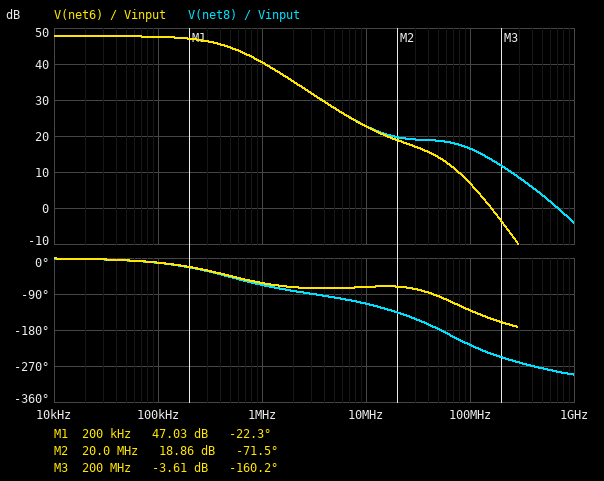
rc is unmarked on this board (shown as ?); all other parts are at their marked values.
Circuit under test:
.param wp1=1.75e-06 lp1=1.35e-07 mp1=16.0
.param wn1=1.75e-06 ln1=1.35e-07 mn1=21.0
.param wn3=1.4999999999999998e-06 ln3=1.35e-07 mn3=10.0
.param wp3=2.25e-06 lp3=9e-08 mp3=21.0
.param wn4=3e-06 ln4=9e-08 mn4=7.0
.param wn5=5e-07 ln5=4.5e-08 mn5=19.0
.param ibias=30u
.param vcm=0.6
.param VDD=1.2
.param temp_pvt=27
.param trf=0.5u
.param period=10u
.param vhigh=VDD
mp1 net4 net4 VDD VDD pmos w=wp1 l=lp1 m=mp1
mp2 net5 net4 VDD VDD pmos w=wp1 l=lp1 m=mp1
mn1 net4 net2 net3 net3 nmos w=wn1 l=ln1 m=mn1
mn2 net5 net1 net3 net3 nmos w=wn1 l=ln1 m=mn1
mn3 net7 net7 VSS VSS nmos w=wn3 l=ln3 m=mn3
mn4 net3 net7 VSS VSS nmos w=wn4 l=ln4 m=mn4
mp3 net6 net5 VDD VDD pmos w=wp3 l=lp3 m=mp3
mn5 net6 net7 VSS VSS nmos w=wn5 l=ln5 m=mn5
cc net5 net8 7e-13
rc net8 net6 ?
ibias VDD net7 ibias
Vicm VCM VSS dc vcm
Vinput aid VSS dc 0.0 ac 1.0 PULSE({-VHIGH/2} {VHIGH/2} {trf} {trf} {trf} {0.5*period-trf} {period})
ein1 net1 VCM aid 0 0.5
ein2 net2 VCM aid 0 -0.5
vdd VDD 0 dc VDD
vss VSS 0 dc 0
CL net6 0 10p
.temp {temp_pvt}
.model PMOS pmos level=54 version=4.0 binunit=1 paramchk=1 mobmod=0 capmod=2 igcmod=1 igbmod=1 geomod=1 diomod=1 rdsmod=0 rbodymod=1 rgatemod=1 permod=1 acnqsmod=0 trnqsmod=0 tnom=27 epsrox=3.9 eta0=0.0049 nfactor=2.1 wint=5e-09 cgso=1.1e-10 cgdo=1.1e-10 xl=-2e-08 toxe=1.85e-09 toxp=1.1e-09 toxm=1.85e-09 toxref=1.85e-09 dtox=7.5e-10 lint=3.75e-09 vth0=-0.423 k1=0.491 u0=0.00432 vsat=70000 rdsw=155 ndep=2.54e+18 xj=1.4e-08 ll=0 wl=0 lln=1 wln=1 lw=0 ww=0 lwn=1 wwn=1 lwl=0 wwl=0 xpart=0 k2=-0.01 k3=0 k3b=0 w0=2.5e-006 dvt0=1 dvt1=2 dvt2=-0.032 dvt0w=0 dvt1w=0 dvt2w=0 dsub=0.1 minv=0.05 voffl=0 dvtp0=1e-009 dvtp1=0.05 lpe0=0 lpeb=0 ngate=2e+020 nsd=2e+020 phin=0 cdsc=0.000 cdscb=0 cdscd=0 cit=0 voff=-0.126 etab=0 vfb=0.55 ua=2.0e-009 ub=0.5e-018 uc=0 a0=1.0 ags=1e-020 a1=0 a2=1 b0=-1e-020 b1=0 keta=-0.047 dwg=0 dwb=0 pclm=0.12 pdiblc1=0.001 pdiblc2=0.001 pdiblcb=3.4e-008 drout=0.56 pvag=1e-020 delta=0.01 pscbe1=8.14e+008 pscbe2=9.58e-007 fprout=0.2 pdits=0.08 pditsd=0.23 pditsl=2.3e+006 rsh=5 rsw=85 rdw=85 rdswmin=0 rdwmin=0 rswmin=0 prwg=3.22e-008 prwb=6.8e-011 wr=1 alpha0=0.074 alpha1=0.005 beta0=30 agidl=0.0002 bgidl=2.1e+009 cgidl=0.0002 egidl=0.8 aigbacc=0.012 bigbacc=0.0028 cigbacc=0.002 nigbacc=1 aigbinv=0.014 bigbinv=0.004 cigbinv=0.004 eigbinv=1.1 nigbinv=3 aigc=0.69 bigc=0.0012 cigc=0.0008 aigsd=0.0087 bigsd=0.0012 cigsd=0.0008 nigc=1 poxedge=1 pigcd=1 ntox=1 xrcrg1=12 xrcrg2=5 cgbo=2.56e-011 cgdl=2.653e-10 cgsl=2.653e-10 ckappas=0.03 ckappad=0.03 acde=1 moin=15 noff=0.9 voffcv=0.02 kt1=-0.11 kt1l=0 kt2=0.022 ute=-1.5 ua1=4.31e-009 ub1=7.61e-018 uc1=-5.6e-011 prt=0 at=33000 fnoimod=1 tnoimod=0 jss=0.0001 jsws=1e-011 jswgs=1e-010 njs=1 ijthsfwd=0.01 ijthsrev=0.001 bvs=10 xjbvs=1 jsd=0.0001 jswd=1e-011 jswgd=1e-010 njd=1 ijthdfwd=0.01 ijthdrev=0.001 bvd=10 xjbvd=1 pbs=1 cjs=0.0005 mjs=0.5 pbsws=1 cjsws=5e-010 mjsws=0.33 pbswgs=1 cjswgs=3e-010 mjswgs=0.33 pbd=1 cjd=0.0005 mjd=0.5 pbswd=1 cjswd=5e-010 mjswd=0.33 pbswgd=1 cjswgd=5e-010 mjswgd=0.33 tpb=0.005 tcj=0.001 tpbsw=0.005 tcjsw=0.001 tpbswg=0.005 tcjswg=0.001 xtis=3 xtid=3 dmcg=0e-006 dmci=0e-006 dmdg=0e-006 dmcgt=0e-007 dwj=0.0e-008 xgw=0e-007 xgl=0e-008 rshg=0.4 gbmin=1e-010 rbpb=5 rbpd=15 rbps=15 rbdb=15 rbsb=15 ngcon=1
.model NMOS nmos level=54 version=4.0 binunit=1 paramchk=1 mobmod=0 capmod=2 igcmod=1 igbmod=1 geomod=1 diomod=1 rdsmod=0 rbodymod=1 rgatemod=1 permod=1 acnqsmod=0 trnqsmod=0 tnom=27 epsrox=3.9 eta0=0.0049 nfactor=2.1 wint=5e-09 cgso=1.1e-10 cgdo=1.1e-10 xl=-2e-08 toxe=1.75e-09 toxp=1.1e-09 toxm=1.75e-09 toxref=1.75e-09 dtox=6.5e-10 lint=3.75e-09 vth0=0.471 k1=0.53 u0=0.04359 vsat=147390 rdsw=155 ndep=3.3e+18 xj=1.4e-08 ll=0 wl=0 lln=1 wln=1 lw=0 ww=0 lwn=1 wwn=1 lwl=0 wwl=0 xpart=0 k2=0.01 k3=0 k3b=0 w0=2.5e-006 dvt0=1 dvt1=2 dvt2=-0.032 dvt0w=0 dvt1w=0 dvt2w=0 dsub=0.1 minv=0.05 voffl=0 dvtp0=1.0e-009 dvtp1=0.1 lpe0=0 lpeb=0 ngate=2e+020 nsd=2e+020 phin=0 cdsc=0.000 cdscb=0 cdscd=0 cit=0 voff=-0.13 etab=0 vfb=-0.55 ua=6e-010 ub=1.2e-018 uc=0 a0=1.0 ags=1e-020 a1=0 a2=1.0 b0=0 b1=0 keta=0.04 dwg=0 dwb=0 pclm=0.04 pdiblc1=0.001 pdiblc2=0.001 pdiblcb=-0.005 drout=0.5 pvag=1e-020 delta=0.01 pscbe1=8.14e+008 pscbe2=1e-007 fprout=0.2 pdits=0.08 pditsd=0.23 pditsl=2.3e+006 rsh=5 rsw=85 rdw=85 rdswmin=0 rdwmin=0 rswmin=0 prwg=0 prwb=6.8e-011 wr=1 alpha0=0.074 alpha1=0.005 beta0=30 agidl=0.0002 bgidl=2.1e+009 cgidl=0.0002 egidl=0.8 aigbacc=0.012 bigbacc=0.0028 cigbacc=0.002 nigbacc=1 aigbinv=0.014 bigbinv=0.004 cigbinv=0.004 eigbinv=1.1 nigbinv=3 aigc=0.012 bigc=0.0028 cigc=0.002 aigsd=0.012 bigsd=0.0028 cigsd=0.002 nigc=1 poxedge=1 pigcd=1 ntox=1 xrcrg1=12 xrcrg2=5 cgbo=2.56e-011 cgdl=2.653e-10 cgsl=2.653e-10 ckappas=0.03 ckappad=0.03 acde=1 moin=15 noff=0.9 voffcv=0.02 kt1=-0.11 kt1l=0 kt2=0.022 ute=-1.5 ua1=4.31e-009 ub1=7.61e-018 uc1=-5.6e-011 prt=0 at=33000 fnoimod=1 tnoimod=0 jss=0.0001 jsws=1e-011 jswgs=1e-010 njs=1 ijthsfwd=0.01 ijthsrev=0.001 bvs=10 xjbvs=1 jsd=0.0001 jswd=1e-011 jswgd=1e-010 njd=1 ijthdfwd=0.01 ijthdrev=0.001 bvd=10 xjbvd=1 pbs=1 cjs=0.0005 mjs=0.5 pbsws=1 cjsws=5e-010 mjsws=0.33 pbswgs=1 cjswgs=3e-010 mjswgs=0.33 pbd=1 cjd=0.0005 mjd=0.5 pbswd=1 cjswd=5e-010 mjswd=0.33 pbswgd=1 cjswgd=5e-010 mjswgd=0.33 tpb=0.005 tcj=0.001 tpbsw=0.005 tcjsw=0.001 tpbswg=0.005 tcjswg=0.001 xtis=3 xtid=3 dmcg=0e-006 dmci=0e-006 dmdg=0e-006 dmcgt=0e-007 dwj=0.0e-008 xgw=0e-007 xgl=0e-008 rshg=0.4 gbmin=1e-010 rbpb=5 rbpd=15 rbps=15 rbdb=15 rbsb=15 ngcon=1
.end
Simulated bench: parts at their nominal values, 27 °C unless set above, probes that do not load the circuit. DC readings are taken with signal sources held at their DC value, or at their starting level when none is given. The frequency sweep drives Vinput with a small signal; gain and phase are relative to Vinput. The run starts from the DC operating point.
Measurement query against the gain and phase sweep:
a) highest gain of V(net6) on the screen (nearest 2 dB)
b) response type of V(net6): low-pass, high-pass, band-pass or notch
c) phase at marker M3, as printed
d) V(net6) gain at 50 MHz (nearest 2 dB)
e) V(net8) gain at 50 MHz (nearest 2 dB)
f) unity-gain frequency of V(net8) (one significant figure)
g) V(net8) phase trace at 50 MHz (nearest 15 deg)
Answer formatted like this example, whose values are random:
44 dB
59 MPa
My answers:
48 dB
low-pass
-160.2 deg
14 dB
18 dB
700 MHz
-180 deg
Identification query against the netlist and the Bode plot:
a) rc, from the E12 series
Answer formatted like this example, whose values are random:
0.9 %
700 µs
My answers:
15 kΩ
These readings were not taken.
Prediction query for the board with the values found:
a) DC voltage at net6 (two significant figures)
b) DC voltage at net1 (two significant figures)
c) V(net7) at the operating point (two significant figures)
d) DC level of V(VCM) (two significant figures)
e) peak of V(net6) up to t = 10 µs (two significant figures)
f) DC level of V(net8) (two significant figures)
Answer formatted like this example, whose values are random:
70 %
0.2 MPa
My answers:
110 mV
600 mV
400 mV
600 mV
1.1 V
110 mV
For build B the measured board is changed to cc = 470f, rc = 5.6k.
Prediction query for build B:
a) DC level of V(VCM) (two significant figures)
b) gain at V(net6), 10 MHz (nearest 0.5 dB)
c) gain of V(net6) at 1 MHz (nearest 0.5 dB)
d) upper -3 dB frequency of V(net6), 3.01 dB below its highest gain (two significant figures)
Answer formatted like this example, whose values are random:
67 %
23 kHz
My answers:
600 mV
24.5 dB
43.0 dB
700 kHz
